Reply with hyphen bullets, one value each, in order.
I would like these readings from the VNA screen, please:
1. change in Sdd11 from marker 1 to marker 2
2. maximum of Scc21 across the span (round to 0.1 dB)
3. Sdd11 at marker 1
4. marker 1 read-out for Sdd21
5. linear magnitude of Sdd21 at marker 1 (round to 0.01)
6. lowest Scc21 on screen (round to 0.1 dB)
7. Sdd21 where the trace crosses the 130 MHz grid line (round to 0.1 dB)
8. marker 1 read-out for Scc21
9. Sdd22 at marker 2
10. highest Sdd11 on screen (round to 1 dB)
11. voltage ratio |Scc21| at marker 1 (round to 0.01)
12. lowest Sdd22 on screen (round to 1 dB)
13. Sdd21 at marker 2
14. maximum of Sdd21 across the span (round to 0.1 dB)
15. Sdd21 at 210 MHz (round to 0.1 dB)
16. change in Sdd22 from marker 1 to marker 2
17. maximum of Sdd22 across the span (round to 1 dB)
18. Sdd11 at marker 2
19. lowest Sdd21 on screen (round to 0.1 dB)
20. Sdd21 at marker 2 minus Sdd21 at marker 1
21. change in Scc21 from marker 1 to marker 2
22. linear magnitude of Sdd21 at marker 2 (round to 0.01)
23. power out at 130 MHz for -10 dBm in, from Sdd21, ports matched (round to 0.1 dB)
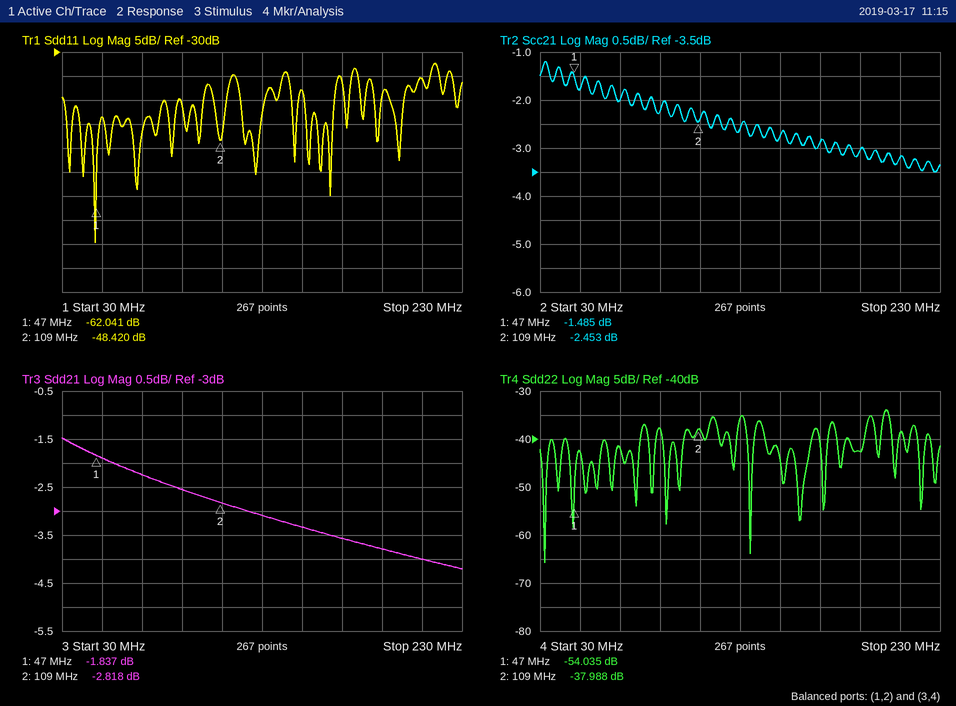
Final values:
- 13.621 dB
- -1.2 dB
- -62.041 dB
- -1.837 dB
- 0.81
- -3.5 dB
- -3.1 dB
- -1.485 dB
- -37.988 dB
- -32 dB
- 0.84
- -66 dB
- -2.818 dB
- -1.5 dB
- -4.0 dB
- 16.047 dB
- -34 dB
- -48.420 dB
- -4.2 dB
- -0.981 dB
- -0.968 dB
- 0.72
- -13.1 dBm
